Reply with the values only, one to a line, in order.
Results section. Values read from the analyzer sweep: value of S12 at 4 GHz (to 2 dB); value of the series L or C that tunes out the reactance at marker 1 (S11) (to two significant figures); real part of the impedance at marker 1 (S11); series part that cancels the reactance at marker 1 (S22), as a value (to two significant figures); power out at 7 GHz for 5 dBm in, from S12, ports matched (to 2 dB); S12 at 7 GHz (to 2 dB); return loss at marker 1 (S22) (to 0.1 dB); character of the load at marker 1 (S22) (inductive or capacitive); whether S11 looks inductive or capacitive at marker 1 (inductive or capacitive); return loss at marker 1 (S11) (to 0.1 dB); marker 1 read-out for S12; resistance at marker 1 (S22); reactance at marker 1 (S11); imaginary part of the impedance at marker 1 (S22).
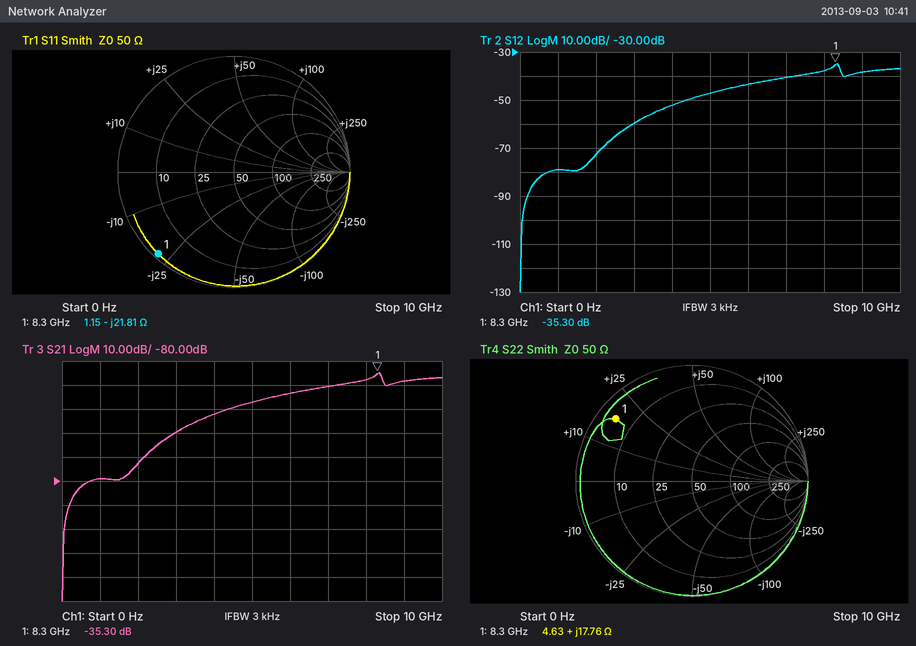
-52 dB
420 pH
1.15 Ω
1.1 pF
-36 dBm
-40 dB
1.4 dB
inductive
capacitive
0.3 dB
-35.30 dB
4.63 Ω
-21.81 Ω
+17.76 Ω
